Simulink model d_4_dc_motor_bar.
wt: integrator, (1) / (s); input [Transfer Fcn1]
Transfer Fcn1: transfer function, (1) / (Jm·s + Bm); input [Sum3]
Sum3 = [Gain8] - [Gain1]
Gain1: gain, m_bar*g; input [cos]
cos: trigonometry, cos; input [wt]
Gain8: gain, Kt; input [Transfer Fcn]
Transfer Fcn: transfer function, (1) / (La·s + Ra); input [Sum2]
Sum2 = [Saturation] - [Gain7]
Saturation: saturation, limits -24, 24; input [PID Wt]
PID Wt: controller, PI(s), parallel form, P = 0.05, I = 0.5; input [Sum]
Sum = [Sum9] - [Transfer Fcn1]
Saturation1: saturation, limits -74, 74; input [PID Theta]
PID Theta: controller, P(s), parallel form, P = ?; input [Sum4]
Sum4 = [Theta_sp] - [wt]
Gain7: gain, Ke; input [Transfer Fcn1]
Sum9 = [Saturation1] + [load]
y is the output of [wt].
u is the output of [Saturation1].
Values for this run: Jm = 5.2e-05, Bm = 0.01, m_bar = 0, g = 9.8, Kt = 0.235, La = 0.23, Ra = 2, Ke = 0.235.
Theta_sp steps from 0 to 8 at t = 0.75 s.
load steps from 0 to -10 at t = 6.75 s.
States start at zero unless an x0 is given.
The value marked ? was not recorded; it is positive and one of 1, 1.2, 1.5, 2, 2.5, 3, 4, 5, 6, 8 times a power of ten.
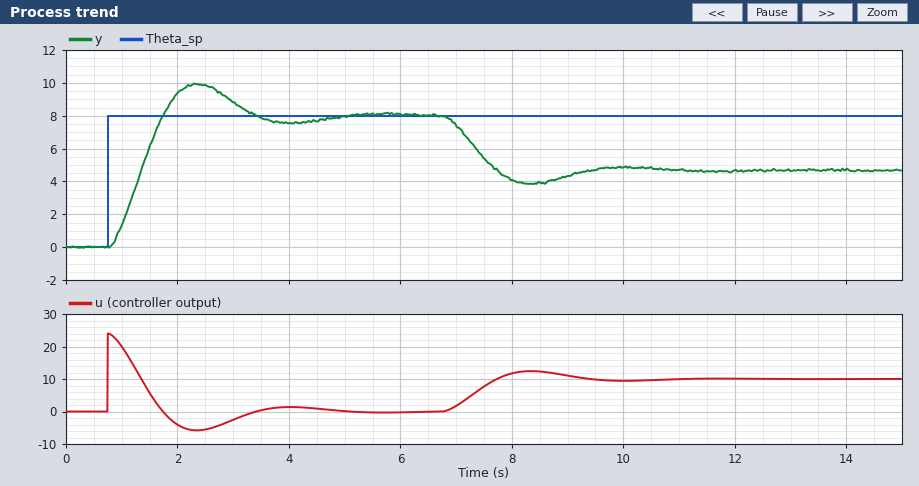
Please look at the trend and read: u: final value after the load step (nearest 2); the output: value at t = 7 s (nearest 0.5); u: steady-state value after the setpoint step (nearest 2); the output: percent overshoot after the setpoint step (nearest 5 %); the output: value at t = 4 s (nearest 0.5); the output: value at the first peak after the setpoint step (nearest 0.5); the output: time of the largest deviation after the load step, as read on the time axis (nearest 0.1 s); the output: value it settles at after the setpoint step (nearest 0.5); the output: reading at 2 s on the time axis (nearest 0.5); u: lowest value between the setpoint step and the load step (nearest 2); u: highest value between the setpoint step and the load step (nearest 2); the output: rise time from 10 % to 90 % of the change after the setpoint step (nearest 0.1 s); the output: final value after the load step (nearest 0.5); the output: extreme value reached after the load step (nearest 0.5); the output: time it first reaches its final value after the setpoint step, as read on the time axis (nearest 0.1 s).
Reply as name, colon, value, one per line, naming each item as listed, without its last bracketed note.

u: final value after the load step: 10
the output: value at t = 7 s: 7.5
u: steady-state value after the setpoint step: 0
the output: percent overshoot after the setpoint step: 25 %
the output: value at t = 4 s: 7.5
the output: value at the first peak after the setpoint step: 10.0
the output: time of the largest deviation after the load step, as read on the time axis: 8.3 s
the output: value it settles at after the setpoint step: 8.0
the output: reading at 2 s on the time axis: 9.5
u: lowest value between the setpoint step and the load step: -6
u: highest value between the setpoint step and the load step: 24
the output: rise time from 10 % to 90 % of the change after the setpoint step: 0.7 s
the output: final value after the load step: 4.5
the output: extreme value reached after the load step: 4.0
the output: time it first reaches its final value after the setpoint step, as read on the time axis: 1.7 s
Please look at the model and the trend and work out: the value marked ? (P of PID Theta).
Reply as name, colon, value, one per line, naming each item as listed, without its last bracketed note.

the value marked ?: 3
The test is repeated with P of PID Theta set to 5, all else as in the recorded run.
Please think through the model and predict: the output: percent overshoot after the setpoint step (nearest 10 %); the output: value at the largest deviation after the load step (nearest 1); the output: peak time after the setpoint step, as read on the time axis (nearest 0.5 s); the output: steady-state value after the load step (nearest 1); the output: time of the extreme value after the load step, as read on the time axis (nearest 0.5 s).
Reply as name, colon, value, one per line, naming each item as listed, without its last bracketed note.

the output: percent overshoot after the setpoint step: 30 %
the output: value at the largest deviation after the load step: 5
the output: peak time after the setpoint step, as read on the time axis: 2.0 s
the output: steady-state value after the load step: 6
the output: time of the extreme value after the load step, as read on the time axis: 8.0 s
